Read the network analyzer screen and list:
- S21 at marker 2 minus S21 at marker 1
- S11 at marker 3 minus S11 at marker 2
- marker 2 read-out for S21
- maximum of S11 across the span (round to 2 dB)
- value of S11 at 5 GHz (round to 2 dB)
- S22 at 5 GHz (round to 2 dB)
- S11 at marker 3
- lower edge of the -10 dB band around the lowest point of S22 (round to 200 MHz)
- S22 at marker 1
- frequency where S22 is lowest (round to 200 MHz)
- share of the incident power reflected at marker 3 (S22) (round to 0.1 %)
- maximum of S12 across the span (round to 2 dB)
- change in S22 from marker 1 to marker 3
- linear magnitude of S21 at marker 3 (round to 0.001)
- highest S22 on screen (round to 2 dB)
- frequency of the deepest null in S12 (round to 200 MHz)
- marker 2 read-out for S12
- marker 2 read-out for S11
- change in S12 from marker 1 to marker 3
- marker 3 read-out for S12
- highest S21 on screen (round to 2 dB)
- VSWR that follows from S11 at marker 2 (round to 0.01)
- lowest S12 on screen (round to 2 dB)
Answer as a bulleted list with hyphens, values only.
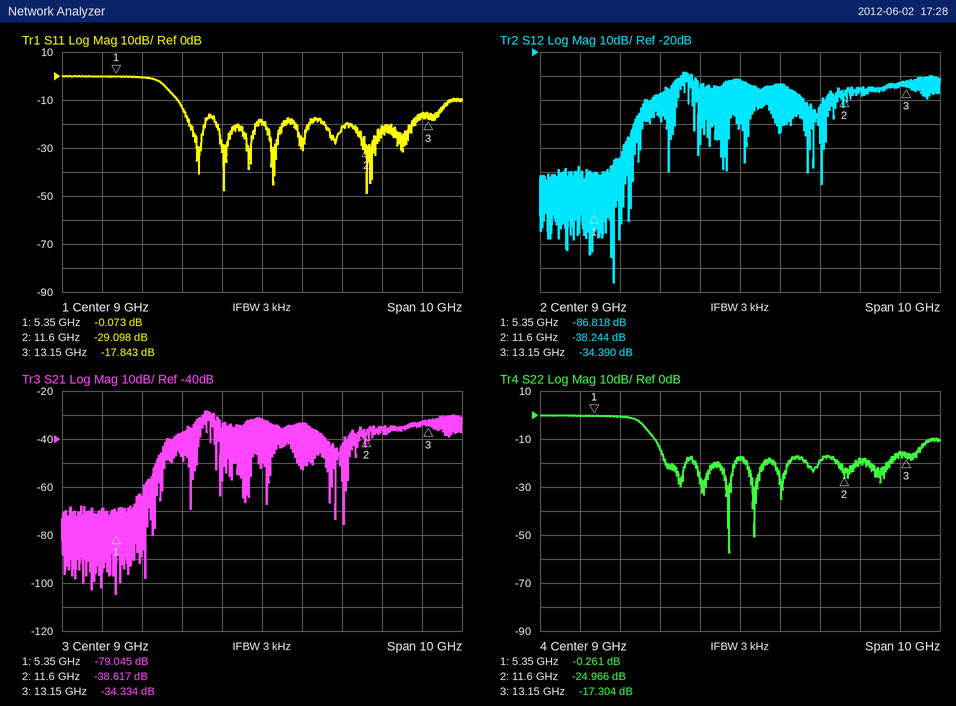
- 40.428 dB
- 11.255 dB
- -38.617 dB
- 0 dB
- 0 dB
- 0 dB
- -17.843 dB
- 6.8 GHz
- -0.261 dB
- 8.8 GHz
- 1.9 %
- -28 dB
- -17.043 dB
- 0.019
- 0 dB
- 5.8 GHz
- -38.244 dB
- -29.098 dB
- 52.428 dB
- -34.390 dB
- -28 dB
- 1.07
- -116 dB
